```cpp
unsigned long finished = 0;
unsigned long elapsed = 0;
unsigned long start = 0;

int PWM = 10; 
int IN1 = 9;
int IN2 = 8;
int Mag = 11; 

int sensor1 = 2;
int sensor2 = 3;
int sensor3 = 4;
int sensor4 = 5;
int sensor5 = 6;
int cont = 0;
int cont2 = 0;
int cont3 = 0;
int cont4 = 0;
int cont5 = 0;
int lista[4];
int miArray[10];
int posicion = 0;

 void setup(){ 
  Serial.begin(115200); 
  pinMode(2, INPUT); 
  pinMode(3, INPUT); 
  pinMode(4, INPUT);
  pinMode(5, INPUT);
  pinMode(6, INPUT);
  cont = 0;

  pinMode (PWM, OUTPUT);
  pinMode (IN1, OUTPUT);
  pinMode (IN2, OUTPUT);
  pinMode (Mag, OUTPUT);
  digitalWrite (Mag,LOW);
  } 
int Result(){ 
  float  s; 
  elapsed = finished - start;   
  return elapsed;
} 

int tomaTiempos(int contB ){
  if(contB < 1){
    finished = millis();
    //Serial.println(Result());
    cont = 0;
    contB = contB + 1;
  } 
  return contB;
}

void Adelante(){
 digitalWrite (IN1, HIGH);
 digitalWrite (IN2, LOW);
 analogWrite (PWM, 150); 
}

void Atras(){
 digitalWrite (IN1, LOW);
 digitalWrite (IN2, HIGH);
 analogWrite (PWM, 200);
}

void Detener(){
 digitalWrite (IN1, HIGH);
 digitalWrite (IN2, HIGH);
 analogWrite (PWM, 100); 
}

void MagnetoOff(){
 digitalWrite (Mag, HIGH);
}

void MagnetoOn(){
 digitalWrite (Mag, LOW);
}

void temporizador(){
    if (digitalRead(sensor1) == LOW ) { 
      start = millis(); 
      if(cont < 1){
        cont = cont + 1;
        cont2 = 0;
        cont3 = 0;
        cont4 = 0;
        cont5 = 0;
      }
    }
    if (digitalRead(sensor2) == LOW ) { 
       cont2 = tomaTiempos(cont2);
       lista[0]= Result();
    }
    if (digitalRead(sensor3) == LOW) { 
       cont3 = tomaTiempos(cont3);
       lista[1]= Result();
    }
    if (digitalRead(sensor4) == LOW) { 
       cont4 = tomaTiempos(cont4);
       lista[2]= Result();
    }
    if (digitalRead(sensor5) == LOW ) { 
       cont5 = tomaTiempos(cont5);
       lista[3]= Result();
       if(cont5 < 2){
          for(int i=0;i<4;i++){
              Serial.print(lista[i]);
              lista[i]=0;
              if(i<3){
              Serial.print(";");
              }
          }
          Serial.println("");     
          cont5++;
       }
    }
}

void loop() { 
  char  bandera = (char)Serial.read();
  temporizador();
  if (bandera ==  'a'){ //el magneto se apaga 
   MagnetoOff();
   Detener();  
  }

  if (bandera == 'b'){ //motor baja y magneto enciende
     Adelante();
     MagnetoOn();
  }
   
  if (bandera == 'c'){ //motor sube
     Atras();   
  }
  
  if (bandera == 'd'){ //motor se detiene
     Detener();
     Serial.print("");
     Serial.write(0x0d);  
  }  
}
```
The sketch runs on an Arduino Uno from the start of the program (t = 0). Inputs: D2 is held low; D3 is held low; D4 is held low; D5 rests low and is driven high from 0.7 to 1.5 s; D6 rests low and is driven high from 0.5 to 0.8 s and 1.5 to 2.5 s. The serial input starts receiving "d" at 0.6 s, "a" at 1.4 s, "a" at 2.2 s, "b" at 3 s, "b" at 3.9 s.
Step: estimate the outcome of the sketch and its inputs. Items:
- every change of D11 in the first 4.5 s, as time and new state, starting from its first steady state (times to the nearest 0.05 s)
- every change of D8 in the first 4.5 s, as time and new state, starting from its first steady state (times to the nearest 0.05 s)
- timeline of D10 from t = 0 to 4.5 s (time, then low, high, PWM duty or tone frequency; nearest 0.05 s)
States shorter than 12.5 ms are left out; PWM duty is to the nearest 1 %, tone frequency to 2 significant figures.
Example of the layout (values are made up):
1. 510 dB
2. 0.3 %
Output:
1. 0 s low; 1.4 s high; 3 s low
2. 0 s low; 0.6 s high; 3 s low
3. 0 s low; 0.6 s PWM 39 %; 3 s PWM 59 %
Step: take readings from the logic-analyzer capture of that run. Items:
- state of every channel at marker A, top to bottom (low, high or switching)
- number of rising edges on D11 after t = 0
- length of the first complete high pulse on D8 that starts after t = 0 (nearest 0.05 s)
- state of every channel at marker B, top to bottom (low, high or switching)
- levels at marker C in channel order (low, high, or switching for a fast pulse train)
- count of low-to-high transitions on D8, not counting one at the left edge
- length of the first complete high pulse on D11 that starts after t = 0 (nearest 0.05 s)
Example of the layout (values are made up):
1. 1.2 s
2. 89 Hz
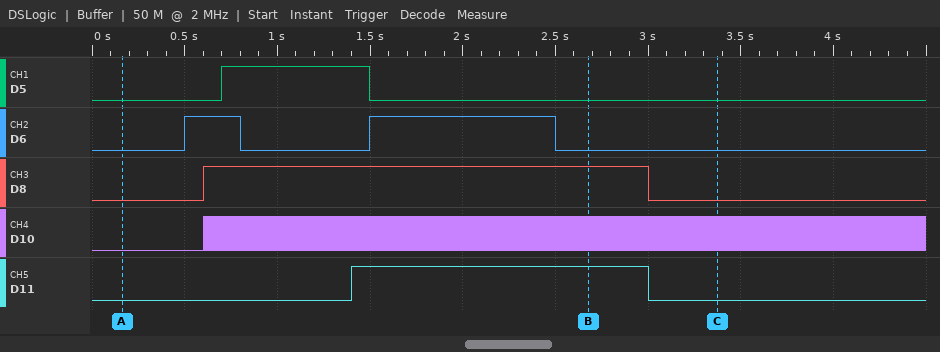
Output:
1. D5 low, D6 low, D8 low, D10 low, D11 low
2. 1
3. 2.40 s
4. D5 low, D6 low, D8 high, D10 switching, D11 high
5. D5 low, D6 low, D8 low, D10 switching, D11 low
6. 1
7. 1.60 s
